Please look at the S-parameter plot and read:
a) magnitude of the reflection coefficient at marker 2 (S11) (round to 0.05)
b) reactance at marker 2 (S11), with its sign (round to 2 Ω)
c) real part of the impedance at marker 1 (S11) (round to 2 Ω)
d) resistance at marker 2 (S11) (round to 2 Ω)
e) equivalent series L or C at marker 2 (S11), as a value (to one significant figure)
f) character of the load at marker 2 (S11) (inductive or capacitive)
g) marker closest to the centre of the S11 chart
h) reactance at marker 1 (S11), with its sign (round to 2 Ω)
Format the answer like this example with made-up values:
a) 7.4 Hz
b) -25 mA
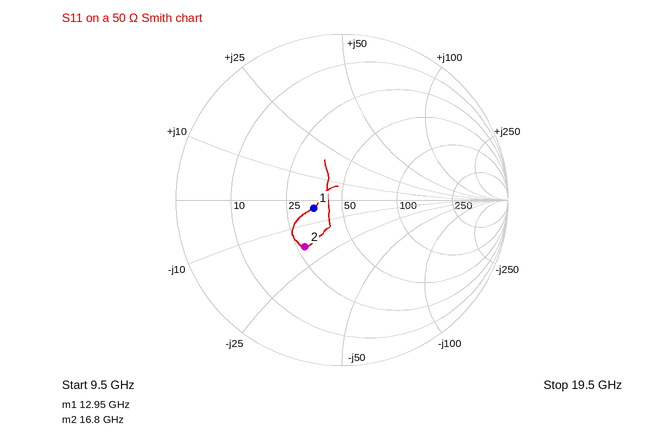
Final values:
a) 0.35
b) -18 Ω
c) 36 Ω
d) 28 Ω
e) 500 fF
f) capacitive
g) marker 1
h) -4 Ω
